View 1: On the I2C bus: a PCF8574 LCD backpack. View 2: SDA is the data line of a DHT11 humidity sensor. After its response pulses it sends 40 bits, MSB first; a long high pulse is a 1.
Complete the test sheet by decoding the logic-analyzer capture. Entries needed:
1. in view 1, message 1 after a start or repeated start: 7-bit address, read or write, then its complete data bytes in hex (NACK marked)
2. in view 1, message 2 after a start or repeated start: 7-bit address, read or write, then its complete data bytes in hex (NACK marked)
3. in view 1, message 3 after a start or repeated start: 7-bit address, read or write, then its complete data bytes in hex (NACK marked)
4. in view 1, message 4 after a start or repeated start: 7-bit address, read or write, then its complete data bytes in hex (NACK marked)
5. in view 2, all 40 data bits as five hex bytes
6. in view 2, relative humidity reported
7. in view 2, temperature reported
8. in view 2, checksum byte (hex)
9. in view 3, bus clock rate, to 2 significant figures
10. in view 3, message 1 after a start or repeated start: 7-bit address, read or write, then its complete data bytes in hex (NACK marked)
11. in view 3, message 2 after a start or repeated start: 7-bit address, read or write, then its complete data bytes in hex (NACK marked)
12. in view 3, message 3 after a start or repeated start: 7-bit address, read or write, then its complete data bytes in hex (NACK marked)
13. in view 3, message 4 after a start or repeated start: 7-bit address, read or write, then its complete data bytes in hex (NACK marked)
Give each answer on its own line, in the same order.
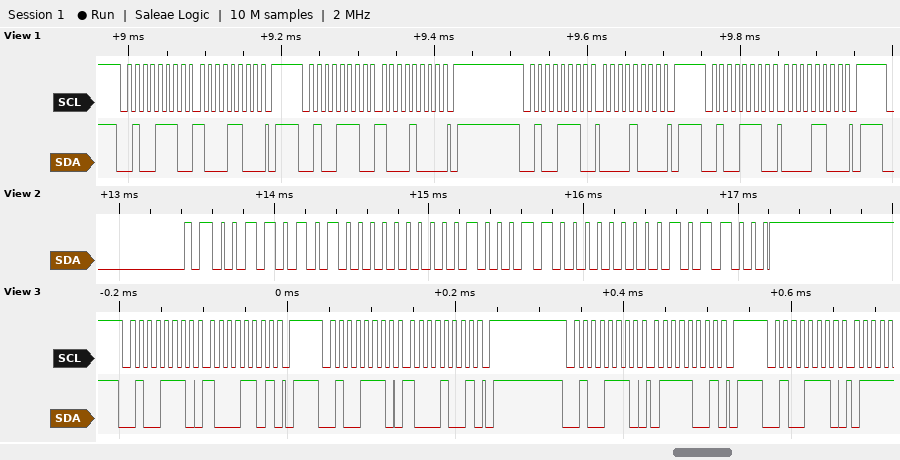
0x27 write: 8C
0x27 write: 88
0x27 write: 08
0x27 write: 0C
35 00 23 00 58
53 %
35.0 °C
0x58
100 kHz
0x27 write: 8D
0x27 write: 89
0x27 write: 79
0x27 write
